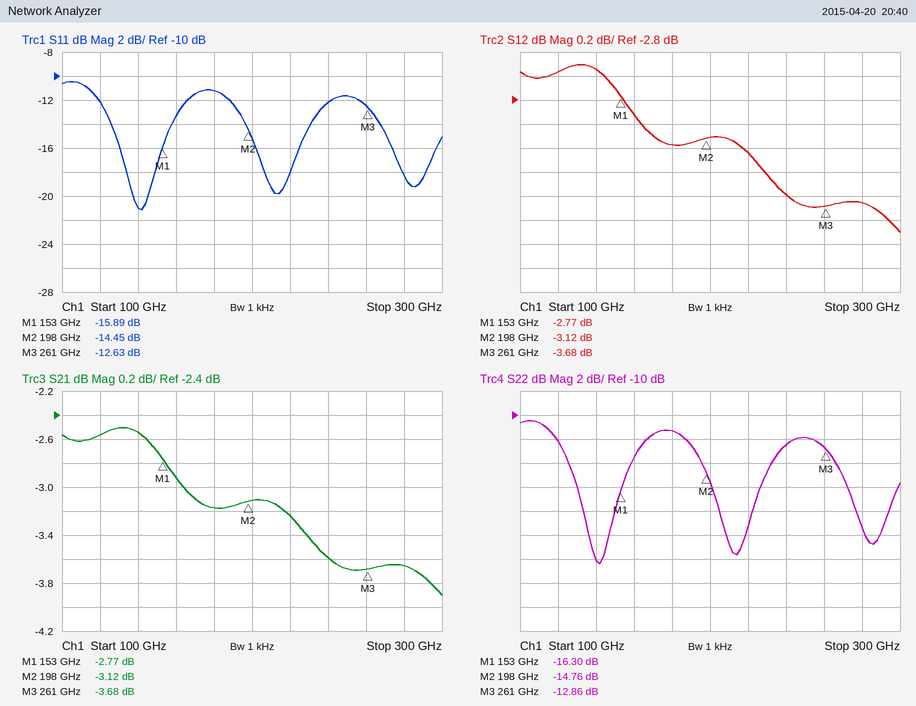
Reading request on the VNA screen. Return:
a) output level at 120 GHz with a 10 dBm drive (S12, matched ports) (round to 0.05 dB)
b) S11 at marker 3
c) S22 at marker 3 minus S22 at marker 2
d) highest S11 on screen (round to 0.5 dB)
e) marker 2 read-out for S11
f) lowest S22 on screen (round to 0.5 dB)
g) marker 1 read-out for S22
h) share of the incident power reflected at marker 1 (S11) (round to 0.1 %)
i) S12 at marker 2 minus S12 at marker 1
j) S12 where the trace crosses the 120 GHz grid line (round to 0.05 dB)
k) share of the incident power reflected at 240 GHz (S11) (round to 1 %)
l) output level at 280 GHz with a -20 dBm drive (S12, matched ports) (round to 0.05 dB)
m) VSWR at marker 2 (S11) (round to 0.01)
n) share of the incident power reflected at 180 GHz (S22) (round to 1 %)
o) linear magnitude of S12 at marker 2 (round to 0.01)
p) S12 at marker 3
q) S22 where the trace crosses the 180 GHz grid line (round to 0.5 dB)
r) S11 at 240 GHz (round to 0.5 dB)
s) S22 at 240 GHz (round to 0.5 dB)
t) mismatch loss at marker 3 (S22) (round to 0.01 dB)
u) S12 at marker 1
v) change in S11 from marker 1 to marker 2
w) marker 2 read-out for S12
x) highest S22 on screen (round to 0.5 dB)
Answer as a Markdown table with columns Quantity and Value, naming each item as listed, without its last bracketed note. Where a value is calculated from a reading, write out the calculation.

| Quantity | Value |
|---|---|
| output level at 120 GHz with a 10 dBm drive (S12, matched ports) | 10 dBm + (-2.55 dB) = 7.45 dBm |
| S11 at marker 3 | -12.63 dB |
| S22 at marker 3 minus S22 at marker 2 | -12.86 − (-14.76) = 1.90 dB |
| highest S11 on screen | -10.5 dB |
| marker 2 read-out for S11 | -14.45 dB |
| lowest S22 on screen | -22.5 dB |
| marker 1 read-out for S22 | -16.30 dB |
| share of the incident power reflected at marker 1 (S11) | 10^(-15.89/10) ≈ 2.6 % |
| S12 at marker 2 minus S12 at marker 1 | -3.12 − (-2.77) = -0.35 dB |
| S12 where the trace crosses the 120 GHz grid line | -2.55 dB |
| share of the incident power reflected at 240 GHz (S11) | 10^(-12/10) ≈ 6 % |
| output level at 280 GHz with a -20 dBm drive (S12, matched ports) | -20 dBm + (-3.65 dB) = -23.65 dBm |
| VSWR at marker 2 (S11) | (1 + 0.1895)/(1 − 0.1895) ≈ 1.47 |
| share of the incident power reflected at 180 GHz (S22) | 10^(-11.5/10) ≈ 7 % |
| linear magnitude of S12 at marker 2 | 10^(-3.12/20) ≈ 0.70 |
| S12 at marker 3 | -3.68 dB |
| S22 where the trace crosses the 180 GHz grid line | -11.5 dB |
| S11 at 240 GHz | -12.0 dB |
| S22 at 240 GHz | -12.5 dB |
| mismatch loss at marker 3 (S22) | −10 log10(1 − 10^(-12.86/10)) ≈ 0.23 dB |
| S12 at marker 1 | -2.77 dB |
| change in S11 from marker 1 to marker 2 | -14.45 − (-15.89) = 1.44 dB |
| marker 2 read-out for S12 | -3.12 dB |
| highest S22 on screen | -10.5 dB |
